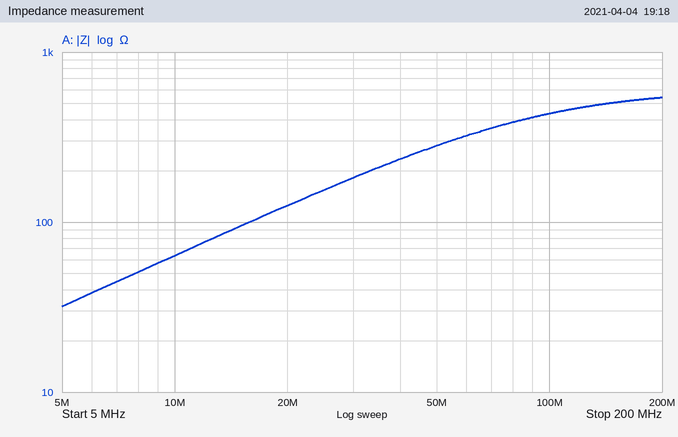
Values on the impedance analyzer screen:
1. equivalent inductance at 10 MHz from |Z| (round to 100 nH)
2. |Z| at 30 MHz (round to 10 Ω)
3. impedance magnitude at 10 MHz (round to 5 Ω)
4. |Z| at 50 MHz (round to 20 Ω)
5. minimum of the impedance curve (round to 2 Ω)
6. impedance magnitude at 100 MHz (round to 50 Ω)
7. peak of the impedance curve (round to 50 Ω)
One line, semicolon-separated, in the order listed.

1.0 µH; 180 Ω; 65 Ω; 280 Ω; 32 Ω; 450 Ω; 550 Ω
